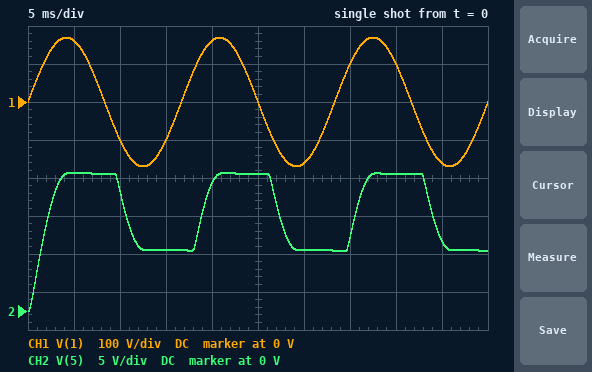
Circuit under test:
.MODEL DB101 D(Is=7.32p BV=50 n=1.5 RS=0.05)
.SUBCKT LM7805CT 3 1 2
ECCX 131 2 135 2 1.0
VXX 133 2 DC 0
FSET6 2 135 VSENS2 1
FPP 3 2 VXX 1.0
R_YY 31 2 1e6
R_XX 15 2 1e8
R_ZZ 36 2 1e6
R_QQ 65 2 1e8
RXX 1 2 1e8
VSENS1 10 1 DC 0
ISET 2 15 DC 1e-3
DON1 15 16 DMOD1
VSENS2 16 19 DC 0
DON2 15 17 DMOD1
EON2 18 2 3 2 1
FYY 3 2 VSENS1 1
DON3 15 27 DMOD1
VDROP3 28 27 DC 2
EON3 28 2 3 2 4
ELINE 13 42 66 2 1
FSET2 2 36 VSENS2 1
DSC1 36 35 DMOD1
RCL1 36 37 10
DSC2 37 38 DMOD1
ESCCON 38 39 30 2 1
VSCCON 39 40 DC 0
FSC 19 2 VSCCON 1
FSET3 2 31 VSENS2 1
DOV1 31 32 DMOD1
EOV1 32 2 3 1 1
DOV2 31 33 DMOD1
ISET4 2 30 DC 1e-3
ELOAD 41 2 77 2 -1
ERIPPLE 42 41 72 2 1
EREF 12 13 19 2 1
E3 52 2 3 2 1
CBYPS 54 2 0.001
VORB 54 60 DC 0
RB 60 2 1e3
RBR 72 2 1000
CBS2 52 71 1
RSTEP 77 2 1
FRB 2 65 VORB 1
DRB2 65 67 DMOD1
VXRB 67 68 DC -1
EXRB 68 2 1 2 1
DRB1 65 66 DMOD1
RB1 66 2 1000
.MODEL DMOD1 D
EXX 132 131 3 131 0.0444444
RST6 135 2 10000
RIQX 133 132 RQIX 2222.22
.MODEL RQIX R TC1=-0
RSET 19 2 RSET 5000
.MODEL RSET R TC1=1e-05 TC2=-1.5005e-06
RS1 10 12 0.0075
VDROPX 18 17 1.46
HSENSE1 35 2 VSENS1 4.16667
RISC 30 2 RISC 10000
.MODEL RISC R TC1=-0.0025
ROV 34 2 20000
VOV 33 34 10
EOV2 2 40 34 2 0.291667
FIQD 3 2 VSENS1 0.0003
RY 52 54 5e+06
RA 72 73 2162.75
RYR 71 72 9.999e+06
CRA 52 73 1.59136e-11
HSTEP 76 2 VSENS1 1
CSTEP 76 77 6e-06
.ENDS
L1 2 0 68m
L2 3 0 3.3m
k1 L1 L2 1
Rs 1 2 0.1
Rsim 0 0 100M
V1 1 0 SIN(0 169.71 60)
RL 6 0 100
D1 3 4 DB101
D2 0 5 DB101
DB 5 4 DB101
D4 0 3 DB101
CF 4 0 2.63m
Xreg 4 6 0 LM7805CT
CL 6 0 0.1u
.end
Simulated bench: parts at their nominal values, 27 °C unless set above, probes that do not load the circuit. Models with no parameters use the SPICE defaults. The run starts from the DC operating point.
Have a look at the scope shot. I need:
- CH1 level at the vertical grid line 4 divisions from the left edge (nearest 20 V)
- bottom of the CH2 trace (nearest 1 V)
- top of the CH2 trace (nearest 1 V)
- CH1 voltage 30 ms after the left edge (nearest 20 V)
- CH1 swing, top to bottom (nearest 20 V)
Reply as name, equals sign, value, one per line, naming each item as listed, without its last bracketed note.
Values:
CH1 level at the vertical grid line 4 divisions from the left edge = 160 V
bottom of the CH2 trace = 0 V
top of the CH2 trace = 18 V
CH1 voltage 30 ms after the left edge = -160 V
CH1 swing, top to bottom = 340 V
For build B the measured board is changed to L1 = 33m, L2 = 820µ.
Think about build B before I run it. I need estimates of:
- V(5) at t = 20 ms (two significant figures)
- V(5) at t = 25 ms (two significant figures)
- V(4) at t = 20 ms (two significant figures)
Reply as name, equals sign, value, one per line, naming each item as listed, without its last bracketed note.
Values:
V(5) at t = 20 ms = 12 V
V(5) at t = 25 ms = 13 V
V(4) at t = 20 ms = 24 V
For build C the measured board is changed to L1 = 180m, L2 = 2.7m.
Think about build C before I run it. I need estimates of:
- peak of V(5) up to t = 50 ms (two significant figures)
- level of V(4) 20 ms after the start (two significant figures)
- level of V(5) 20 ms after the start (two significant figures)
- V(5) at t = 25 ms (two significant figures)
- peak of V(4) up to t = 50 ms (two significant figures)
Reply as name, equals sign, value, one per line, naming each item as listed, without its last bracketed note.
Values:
peak of V(5) up to t = 50 ms = 9.9 V
level of V(4) 20 ms after the start = 19 V
level of V(5) 20 ms after the start = 9.7 V
V(5) at t = 25 ms = 9.8 V
peak of V(4) up to t = 50 ms = 20 V
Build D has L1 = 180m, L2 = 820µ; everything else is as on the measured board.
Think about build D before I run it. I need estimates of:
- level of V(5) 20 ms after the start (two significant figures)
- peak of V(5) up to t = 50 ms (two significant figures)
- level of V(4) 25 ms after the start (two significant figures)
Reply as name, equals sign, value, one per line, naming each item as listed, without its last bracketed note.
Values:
level of V(5) 20 ms after the start = 5.1 V
peak of V(5) up to t = 50 ms = 5.2 V
level of V(4) 25 ms after the start = 10 V
